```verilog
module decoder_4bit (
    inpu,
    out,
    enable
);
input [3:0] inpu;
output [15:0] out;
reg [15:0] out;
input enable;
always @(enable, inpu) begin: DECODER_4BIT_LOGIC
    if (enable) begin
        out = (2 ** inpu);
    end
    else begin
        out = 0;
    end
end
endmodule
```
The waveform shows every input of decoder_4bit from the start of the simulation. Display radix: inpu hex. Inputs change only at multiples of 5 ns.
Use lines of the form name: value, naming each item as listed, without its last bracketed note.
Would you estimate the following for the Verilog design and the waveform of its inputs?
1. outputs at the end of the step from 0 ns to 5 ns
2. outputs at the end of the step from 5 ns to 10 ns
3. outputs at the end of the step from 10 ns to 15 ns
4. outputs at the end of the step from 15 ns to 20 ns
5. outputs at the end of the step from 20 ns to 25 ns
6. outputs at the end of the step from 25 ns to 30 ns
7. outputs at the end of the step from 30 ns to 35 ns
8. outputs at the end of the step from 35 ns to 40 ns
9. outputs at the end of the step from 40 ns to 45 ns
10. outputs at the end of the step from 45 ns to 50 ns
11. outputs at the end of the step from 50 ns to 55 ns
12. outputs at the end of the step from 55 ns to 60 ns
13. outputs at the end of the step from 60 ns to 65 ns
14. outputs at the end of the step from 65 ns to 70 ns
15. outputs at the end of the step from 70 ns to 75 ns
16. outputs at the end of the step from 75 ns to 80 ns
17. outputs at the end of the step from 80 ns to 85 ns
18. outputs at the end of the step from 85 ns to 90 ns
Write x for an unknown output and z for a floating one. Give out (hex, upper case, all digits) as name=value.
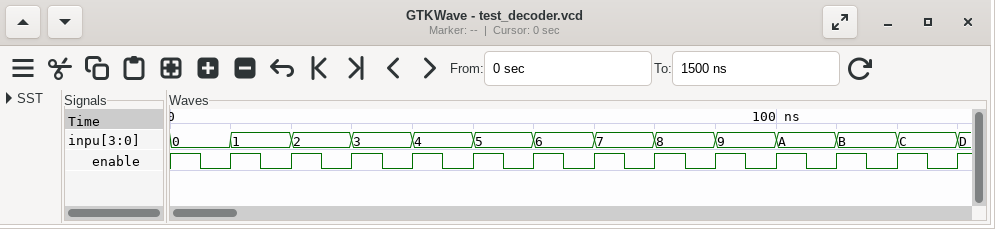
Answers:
outputs at the end of the step from 0 ns to 5 ns: out=0001
outputs at the end of the step from 5 ns to 10 ns: out=0000
outputs at the end of the step from 10 ns to 15 ns: out=0002
outputs at the end of the step from 15 ns to 20 ns: out=0000
outputs at the end of the step from 20 ns to 25 ns: out=0004
outputs at the end of the step from 25 ns to 30 ns: out=0000
outputs at the end of the step from 30 ns to 35 ns: out=0008
outputs at the end of the step from 35 ns to 40 ns: out=0000
outputs at the end of the step from 40 ns to 45 ns: out=0010
outputs at the end of the step from 45 ns to 50 ns: out=0000
outputs at the end of the step from 50 ns to 55 ns: out=0020
outputs at the end of the step from 55 ns to 60 ns: out=0000
outputs at the end of the step from 60 ns to 65 ns: out=0040
outputs at the end of the step from 65 ns to 70 ns: out=0000
outputs at the end of the step from 70 ns to 75 ns: out=0080
outputs at the end of the step from 75 ns to 80 ns: out=0000
outputs at the end of the step from 80 ns to 85 ns: out=0100
outputs at the end of the step from 85 ns to 90 ns: out=0000
